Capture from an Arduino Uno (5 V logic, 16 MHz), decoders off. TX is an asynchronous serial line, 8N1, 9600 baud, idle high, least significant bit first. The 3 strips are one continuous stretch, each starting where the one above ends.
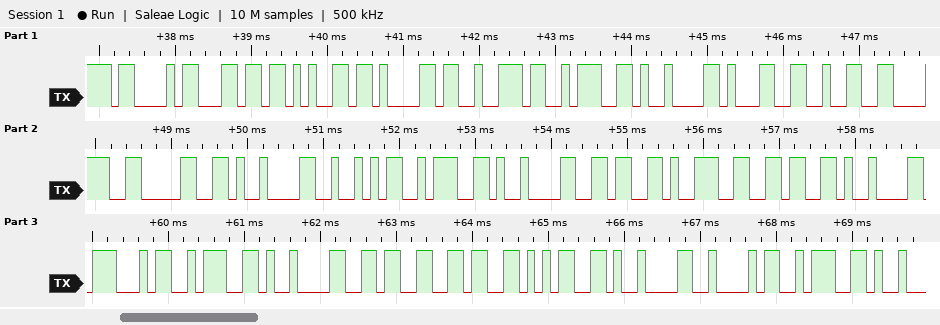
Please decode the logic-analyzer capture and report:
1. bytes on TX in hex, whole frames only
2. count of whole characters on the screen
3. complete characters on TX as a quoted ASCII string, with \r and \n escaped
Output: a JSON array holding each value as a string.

["0x43 0x6C 0x65 0x61 0x72 0x3A 0x09 0x31 0x32 0x38 0x30 0x09 0x52 0x3A 0x09 0x36 0x39 0x36 0x09 0x47 0x3A 0x09 0x36 0x36 0x35 0x09 0x42 0x3A", "28", "\"Clear:\\t1280\\tR:\\t696\\tG:\\t665\\tB:\""]
